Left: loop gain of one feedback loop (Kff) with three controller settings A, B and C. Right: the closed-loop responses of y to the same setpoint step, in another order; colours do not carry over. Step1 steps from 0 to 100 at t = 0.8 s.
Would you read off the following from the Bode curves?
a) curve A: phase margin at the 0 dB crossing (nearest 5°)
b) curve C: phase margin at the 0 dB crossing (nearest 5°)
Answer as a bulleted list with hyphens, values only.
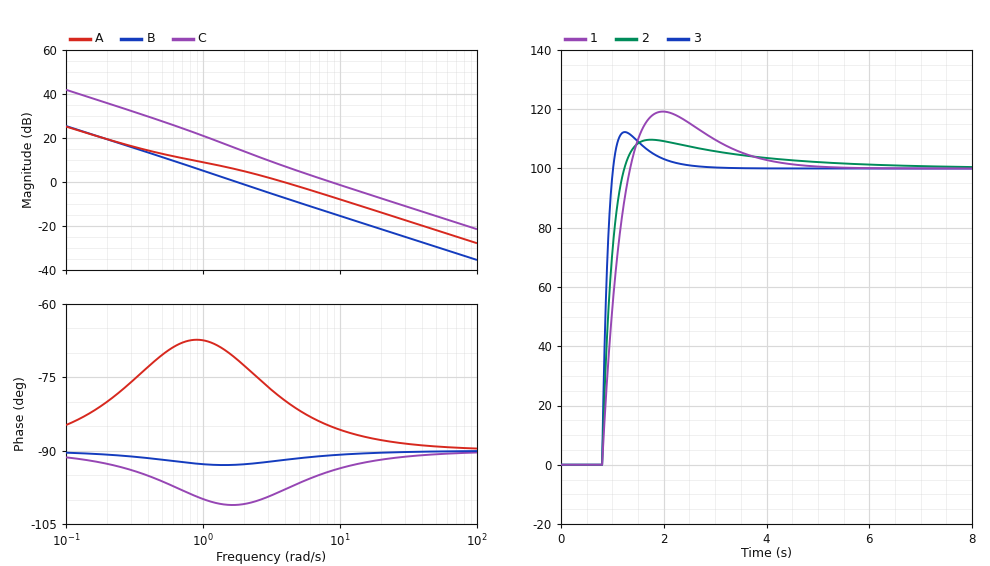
- 100°
- 85°
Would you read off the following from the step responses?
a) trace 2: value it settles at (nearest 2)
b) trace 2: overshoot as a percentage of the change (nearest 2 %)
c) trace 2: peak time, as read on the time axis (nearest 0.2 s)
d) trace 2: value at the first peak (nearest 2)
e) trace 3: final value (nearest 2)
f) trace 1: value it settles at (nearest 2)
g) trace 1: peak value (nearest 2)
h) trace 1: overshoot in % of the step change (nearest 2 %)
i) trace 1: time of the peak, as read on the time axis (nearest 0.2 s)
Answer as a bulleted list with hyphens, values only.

- 100
- 10 %
- 1.8 s
- 110
- 100
- 100
- 120
- 20 %
- 2.0 s
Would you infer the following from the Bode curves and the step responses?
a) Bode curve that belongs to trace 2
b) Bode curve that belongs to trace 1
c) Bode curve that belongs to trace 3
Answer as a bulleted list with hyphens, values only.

- A
- B
- C
